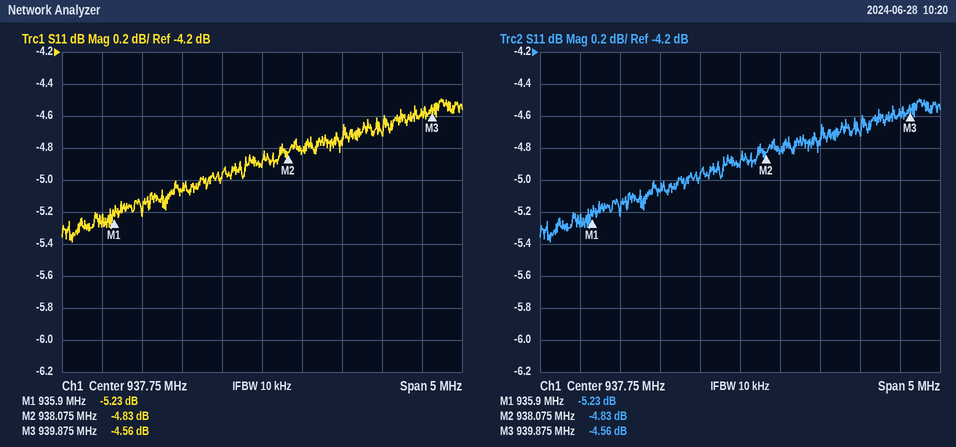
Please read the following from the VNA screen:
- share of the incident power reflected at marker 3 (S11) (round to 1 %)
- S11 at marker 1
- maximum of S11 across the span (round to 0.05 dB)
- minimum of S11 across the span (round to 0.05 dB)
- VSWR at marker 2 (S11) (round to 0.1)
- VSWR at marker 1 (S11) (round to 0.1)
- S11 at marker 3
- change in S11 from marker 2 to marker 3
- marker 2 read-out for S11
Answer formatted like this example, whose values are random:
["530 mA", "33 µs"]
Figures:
["35 %", "-5.23 dB", "-4.50 dB", "-5.40 dB", "3.7", "3.4", "-4.56 dB", "0.27 dB", "-4.83 dB"]
